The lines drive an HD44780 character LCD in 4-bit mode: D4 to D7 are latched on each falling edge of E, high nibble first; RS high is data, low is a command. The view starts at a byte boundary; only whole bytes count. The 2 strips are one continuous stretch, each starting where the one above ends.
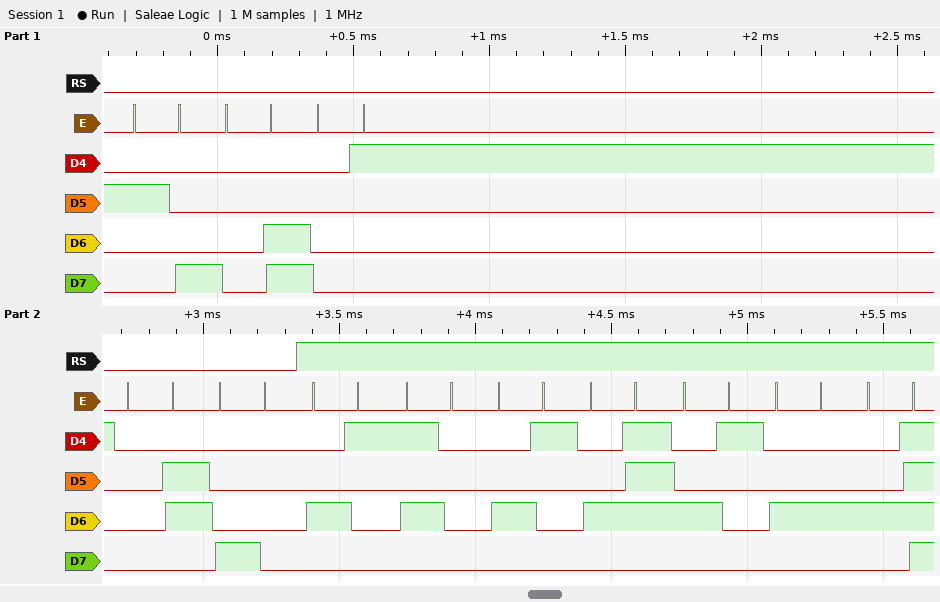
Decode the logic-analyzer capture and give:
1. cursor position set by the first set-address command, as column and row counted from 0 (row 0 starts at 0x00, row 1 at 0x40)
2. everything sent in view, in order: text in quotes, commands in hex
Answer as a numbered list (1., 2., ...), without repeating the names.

1. column 0, row 0
2. 0x28 0x0C 0x01 0x06 0x80 "APAGADO"
